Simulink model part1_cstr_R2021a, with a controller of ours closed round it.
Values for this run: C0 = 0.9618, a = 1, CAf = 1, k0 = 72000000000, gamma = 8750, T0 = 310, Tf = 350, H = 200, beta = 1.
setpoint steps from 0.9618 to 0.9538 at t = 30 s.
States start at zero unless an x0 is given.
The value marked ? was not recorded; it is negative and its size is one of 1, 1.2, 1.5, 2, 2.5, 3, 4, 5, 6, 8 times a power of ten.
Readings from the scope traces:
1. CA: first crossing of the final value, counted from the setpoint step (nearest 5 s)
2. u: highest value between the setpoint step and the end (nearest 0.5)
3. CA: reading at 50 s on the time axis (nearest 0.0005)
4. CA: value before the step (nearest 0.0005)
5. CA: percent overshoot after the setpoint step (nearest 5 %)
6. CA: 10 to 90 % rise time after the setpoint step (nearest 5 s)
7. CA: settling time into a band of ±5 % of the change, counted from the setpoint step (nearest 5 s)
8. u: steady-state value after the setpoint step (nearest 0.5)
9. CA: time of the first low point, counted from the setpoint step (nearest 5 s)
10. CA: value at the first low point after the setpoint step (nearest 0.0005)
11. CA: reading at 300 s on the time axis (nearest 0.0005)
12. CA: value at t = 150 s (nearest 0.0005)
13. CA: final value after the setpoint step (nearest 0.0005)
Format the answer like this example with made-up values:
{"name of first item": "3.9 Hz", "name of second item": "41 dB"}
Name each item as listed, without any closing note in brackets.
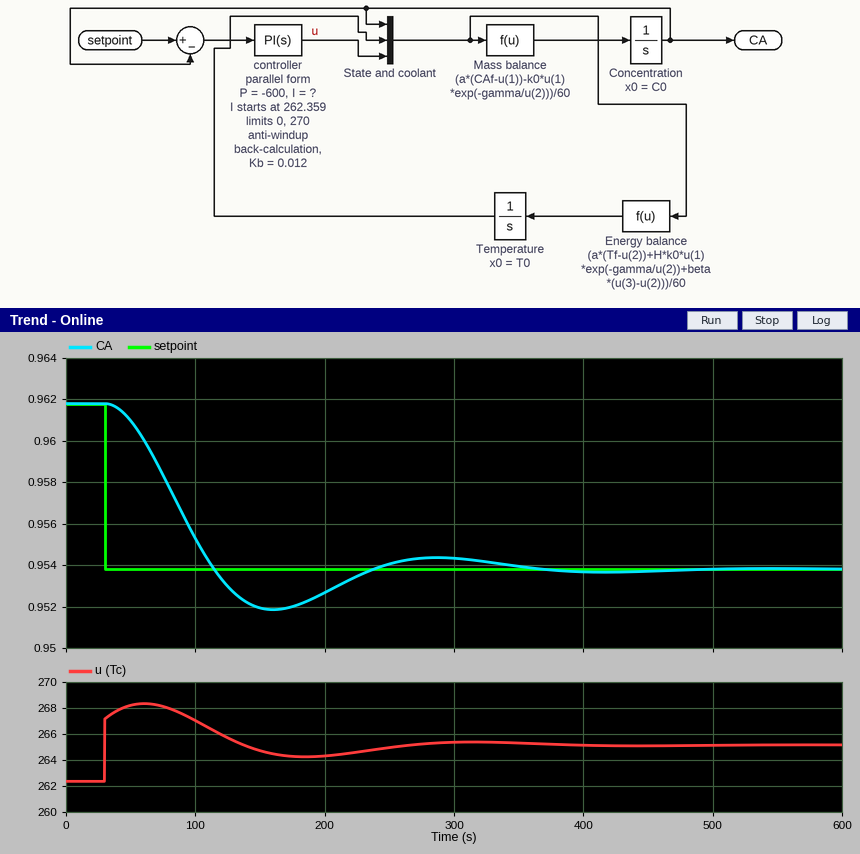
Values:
{"CA: first crossing of the final value, counted from the setpoint step": "85 s", "u: highest value between the setpoint step and the end": "268.5", "CA: reading at 50 s on the time axis": "0.9610", "CA: value before the step": "0.9620", "CA: percent overshoot after the setpoint step": "25 %", "CA: 10 to 90 % rise time after the setpoint step": "55 s", "CA: settling time into a band of ±5 % of the change, counted from the setpoint step": "290 s", "u: steady-state value after the setpoint step": "265.0", "CA: time of the first low point, counted from the setpoint step": "130 s", "CA: value at the first low point after the setpoint step": "0.9520", "CA: reading at 300 s on the time axis": "0.9545", "CA: value at t = 150 s": "0.9520", "CA: final value after the setpoint step": "0.9540"}
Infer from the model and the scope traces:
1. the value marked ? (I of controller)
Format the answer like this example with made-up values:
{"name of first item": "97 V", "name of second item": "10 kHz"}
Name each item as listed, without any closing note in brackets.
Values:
{"the value marked ?": "-10"}
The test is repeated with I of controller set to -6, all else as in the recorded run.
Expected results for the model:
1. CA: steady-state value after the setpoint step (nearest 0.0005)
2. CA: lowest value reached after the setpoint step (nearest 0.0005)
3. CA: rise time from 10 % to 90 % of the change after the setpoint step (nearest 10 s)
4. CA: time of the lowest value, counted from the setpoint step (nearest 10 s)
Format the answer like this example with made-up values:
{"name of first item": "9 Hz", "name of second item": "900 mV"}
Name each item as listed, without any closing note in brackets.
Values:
{"CA: steady-state value after the setpoint step": "0.9540", "CA: lowest value reached after the setpoint step": "0.9535", "CA: rise time from 10 % to 90 % of the change after the setpoint step": "70 s", "CA: time of the lowest value, counted from the setpoint step": "140 s"}
